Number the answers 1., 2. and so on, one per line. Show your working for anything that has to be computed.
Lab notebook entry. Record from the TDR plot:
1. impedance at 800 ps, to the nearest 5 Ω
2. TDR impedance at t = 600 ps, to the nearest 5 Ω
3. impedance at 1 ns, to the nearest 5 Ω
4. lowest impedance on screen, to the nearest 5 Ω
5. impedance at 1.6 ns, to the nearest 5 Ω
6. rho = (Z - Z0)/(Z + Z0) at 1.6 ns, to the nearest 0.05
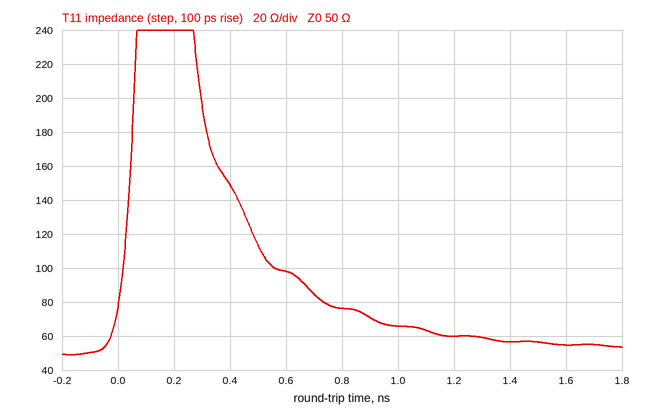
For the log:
1. 75 Ω
2. 100 Ω
3. 65 Ω
4. 50 Ω
5. 55 Ω
6. (55 − 50)/(55 + 50) ≈ +0.05
